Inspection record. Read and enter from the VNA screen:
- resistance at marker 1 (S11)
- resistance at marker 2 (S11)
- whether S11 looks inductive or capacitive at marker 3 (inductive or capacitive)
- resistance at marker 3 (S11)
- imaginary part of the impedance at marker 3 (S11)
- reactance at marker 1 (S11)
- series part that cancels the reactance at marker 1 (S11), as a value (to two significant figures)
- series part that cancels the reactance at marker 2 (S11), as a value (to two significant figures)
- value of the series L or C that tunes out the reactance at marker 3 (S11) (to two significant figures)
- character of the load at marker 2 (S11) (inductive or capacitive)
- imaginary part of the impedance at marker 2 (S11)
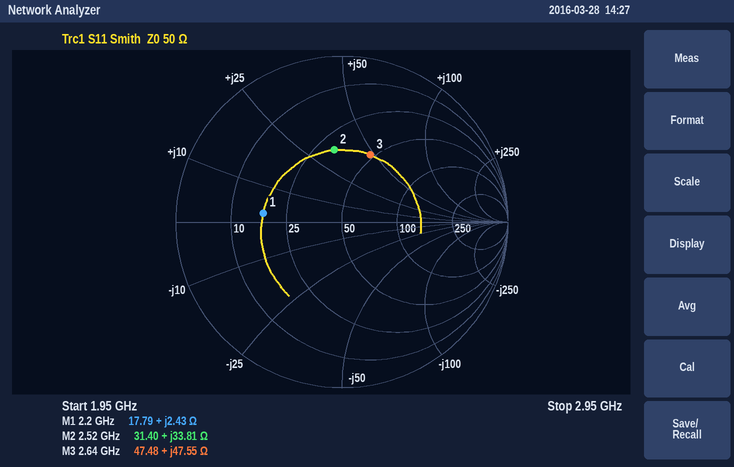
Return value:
17.79 Ω
31.40 Ω
inductive
47.48 Ω
+47.55 Ω
+2.43 Ω
30 pF
1.9 pF
1.3 pF
inductive
+33.81 Ω
